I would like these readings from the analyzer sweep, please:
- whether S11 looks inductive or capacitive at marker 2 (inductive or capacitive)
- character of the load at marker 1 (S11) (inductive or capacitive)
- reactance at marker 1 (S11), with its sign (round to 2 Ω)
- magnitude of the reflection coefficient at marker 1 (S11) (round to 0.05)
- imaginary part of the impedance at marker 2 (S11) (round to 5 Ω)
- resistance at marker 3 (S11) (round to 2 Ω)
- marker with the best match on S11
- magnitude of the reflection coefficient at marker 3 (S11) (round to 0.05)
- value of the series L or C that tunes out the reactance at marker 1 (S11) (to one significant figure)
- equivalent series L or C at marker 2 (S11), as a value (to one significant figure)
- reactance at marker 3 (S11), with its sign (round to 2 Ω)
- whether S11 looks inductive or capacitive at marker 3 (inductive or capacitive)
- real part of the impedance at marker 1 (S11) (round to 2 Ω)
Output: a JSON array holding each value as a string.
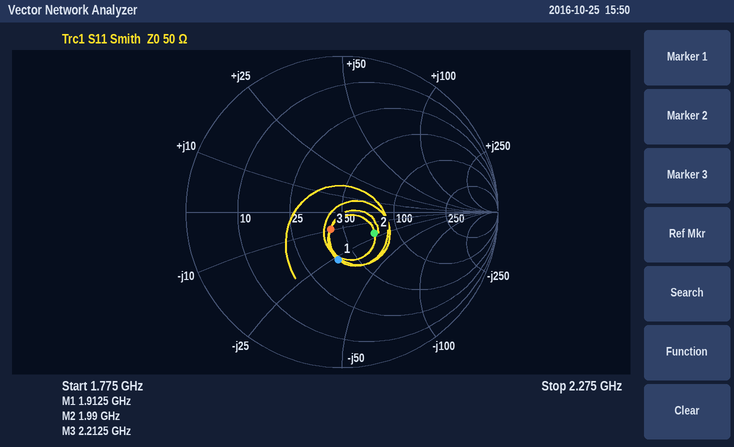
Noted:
["capacitive", "capacitive", "-26 Ω", "0.30", "-20 Ω", "42 Ω", "marker 3", "0.15", "2 nH", "4 pF", "-10 Ω", "capacitive", "40 Ω"]
